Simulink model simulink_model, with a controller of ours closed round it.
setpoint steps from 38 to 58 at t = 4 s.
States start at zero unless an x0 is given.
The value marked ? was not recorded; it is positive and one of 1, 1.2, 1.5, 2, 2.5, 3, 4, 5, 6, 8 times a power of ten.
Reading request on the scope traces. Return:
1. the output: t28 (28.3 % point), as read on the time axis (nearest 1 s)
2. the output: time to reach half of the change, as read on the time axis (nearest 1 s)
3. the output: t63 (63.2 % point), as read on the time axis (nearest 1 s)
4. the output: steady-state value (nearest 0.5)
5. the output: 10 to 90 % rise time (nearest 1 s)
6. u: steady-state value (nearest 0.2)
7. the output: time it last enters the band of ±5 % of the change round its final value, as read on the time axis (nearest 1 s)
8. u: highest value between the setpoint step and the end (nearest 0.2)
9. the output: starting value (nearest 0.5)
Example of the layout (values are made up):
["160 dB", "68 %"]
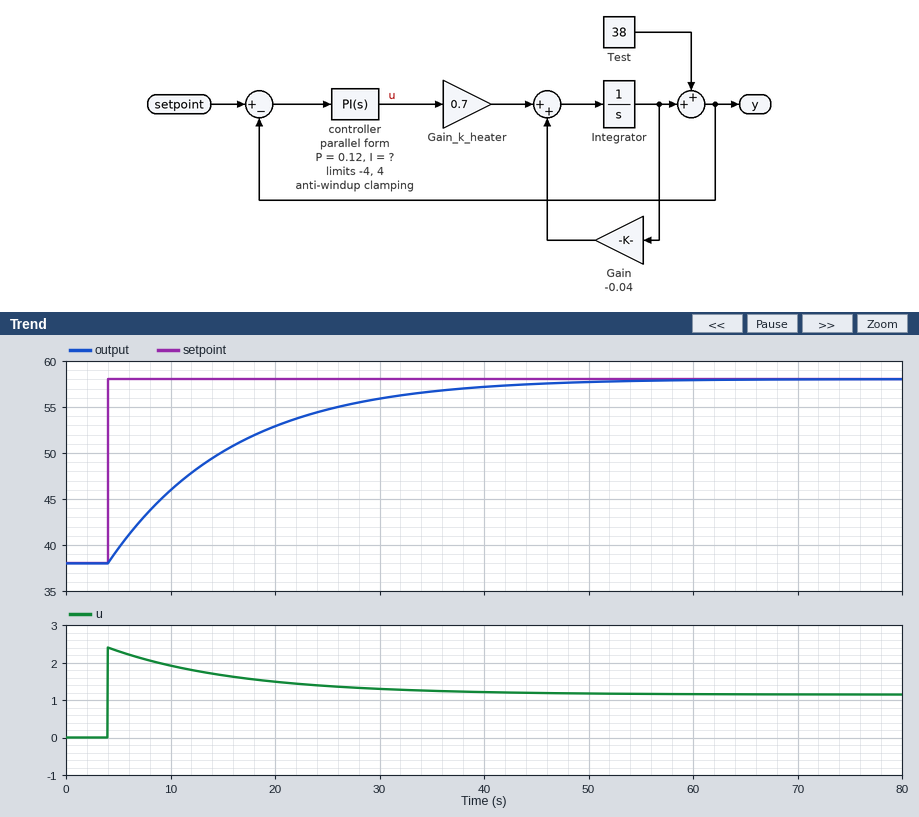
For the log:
["8 s", "12 s", "16 s", "58.0", "25 s", "1.2", "38 s", "2.4", "38.0"]
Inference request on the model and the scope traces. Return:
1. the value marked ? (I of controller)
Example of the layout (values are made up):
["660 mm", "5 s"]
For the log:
["0.005"]
